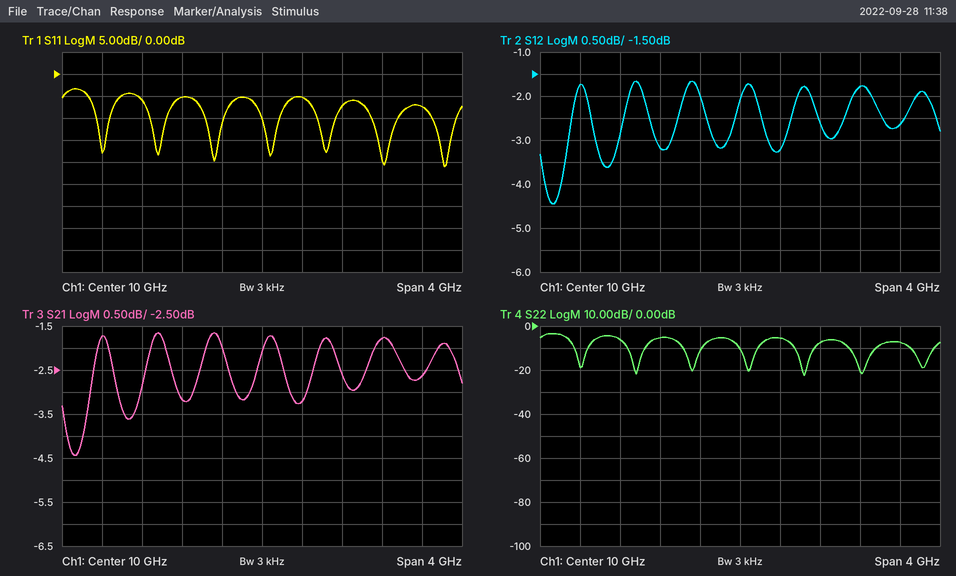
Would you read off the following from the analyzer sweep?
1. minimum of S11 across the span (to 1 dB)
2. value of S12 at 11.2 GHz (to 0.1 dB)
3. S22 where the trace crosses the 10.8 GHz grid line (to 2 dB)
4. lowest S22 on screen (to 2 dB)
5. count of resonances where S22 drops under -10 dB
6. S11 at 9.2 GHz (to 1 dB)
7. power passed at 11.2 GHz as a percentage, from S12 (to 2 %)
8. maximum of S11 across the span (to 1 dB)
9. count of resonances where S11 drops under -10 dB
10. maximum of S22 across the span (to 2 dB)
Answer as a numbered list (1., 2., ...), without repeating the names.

1. -21 dB
2. -1.8 dB
3. -8 dB
4. -22 dB
5. 7
6. -5 dB
7. 66 %
8. -3 dB
9. 7
10. -4 dB
